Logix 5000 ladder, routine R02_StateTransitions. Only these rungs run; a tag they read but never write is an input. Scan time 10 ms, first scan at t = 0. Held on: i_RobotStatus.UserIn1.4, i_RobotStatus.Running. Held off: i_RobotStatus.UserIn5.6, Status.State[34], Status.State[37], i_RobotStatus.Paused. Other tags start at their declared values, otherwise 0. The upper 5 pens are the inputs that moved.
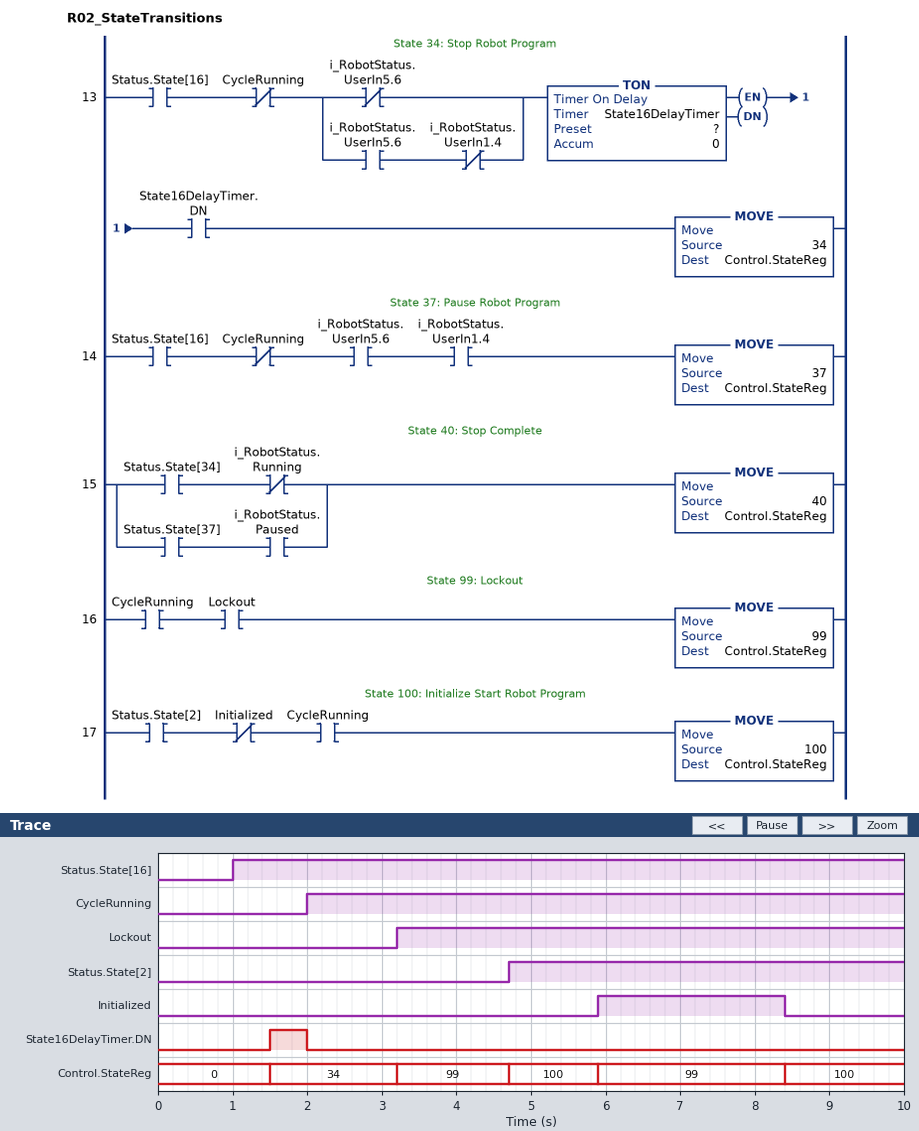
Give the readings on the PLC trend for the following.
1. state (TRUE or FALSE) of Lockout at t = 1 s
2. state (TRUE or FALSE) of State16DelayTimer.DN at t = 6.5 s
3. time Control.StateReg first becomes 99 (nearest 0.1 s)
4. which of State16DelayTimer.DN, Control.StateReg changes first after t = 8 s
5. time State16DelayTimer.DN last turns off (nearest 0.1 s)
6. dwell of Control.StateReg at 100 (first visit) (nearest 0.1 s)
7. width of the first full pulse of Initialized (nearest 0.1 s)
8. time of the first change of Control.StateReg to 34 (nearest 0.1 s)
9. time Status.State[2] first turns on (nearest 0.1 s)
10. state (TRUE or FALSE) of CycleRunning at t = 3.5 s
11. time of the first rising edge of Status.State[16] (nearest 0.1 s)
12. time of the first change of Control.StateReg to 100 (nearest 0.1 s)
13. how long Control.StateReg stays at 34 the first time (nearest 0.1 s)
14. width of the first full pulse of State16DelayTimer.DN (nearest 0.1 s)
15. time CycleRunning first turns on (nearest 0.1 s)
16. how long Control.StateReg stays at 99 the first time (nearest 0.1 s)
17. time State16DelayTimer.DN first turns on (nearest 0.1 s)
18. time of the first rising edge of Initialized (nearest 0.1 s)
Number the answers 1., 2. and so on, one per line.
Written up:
1. FALSE
2. FALSE
3. 3.2 s
4. Control.StateReg
5. 2.0 s
6. 1.2 s
7. 2.5 s
8. 1.5 s
9. 4.7 s
10. TRUE
11. 1.0 s
12. 4.7 s
13. 1.7 s
14. 0.5 s
15. 2.0 s
16. 1.5 s
17. 1.5 s
18. 5.9 s
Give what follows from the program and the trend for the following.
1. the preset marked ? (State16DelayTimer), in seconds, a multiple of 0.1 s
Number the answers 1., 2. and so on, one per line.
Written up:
1. 0.5 s
